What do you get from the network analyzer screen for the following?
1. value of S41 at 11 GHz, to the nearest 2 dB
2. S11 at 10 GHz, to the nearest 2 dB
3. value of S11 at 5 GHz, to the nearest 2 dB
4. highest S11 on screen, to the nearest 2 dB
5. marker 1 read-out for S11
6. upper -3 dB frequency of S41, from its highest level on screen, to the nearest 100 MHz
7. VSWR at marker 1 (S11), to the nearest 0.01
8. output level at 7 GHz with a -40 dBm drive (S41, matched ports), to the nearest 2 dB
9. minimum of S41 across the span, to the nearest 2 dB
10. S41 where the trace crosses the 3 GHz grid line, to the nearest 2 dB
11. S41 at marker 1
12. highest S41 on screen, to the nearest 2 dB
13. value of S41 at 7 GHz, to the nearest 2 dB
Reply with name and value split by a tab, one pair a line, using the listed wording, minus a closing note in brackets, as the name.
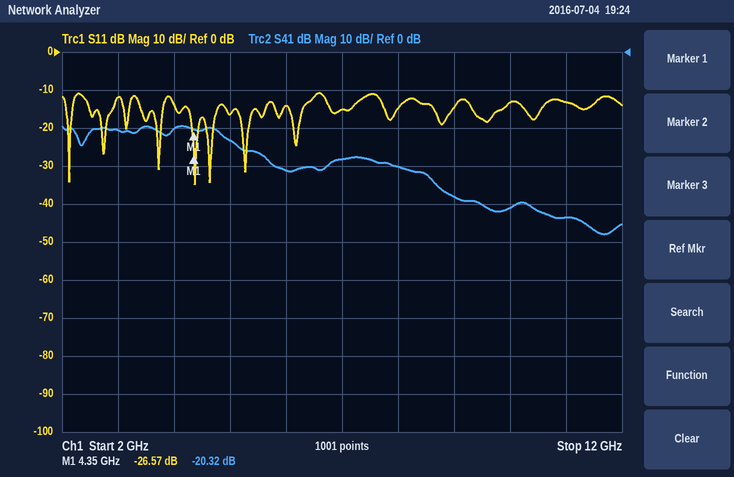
value of S41 at 11 GHz, to the nearest 2 dB	-44 dB
S11 at 10 GHz, to the nearest 2 dB	-14 dB
value of S11 at 5 GHz, to the nearest 2 dB	-16 dB
highest S11 on screen, to the nearest 2 dB	-10 dB
marker 1 read-out for S11	-26.57 dB
upper -3 dB frequency of S41, from its highest level on screen, to the nearest 100 MHz	4.9 GHz
VSWR at marker 1 (S11), to the nearest 0.01	1.10
output level at 7 GHz with a -40 dBm drive (S41, matched ports), to the nearest 2 dB	-68 dBm
minimum of S41 across the span, to the nearest 2 dB	-48 dB
S41 where the trace crosses the 3 GHz grid line, to the nearest 2 dB	-20 dB
S41 at marker 1	-20.32 dB
highest S41 on screen, to the nearest 2 dB	-20 dB
value of S41 at 7 GHz, to the nearest 2 dB	-28 dB
